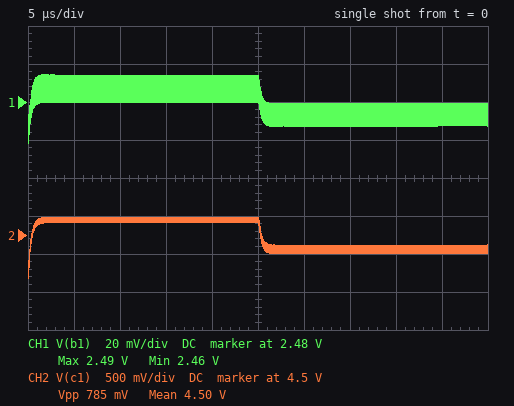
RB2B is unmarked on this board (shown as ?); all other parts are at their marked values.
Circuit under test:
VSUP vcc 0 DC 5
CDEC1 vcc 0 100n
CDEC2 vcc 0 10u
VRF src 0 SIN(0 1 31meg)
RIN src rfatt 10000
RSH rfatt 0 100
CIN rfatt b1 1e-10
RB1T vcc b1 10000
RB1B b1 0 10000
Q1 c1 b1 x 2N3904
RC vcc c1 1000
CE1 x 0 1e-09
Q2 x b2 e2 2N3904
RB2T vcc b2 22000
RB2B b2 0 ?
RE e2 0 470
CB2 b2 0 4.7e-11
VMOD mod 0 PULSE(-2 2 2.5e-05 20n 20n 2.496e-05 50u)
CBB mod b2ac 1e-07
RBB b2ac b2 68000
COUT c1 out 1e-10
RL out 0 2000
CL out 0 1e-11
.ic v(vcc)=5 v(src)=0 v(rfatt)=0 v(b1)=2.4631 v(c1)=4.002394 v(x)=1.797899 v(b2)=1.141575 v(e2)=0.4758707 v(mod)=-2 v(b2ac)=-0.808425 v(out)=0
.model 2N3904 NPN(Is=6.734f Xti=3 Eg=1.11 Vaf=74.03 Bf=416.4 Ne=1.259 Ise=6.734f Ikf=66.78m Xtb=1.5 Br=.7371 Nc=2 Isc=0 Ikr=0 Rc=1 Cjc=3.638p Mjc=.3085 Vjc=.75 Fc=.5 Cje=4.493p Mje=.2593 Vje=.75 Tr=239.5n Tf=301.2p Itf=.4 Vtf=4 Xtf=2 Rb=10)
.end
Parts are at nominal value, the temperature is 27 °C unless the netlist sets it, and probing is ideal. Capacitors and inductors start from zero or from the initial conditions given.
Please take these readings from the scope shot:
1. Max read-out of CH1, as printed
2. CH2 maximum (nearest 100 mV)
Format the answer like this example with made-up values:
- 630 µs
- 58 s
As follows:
- 2.49 V
- 4.7 V
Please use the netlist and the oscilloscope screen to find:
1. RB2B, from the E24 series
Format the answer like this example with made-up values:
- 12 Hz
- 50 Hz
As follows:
- 4.7 kΩ
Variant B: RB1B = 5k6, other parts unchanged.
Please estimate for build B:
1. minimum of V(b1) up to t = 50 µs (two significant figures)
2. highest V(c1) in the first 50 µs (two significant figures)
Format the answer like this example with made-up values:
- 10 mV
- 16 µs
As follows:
- 1.8 V
- 5.0 V
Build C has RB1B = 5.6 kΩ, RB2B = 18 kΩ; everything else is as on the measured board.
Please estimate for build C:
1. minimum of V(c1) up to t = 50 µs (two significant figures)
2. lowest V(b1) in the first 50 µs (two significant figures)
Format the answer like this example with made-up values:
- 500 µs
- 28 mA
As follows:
- 3.0 V
- 1.7 V
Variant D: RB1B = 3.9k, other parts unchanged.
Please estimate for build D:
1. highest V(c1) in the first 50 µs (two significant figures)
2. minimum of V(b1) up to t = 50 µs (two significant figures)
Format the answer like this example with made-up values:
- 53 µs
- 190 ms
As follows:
- 5.0 V
- 1.4 V
